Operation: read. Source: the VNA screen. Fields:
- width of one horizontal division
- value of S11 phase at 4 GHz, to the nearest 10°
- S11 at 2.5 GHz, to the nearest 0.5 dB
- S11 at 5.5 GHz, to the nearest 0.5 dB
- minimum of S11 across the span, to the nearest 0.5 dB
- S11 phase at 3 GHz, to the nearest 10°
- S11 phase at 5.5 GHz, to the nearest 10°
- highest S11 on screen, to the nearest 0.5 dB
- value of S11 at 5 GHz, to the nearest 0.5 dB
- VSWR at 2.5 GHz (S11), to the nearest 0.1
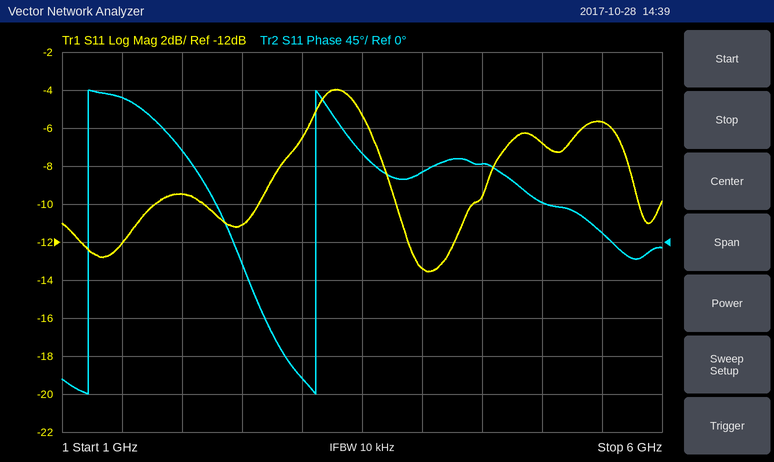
500 MHz
80°
-11.0 dB
-5.5 dB
-13.5 dB
-160°
10°
-4.0 dB
-7.0 dB
1.8
